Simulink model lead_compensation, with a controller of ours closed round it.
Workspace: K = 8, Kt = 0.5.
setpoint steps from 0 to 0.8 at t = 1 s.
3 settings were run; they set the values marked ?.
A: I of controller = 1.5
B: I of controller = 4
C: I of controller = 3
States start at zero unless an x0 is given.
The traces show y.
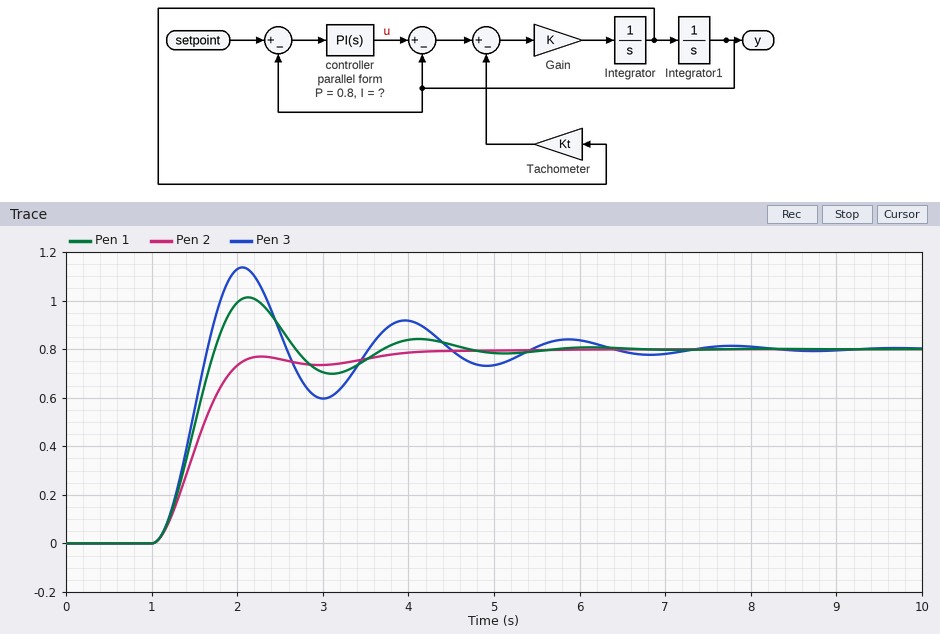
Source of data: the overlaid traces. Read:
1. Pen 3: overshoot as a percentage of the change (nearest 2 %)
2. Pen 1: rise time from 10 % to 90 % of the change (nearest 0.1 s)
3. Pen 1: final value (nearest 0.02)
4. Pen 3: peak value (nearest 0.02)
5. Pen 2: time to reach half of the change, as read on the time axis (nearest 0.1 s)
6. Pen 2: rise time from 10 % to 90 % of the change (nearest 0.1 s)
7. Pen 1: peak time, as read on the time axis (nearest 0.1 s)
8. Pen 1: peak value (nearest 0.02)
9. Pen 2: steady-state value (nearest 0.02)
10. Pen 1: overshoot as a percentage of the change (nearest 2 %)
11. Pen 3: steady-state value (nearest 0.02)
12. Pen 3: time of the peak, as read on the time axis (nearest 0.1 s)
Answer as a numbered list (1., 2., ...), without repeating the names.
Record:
1. 42 %
2. 0.5 s
3. 0.80
4. 1.14
5. 1.5 s
6. 0.8 s
7. 2.1 s
8. 1.02
9. 0.80
10. 26 %
11. 0.80
12. 2.1 s
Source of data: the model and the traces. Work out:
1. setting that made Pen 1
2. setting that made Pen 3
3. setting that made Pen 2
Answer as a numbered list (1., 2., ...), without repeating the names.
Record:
1. C
2. B
3. A
